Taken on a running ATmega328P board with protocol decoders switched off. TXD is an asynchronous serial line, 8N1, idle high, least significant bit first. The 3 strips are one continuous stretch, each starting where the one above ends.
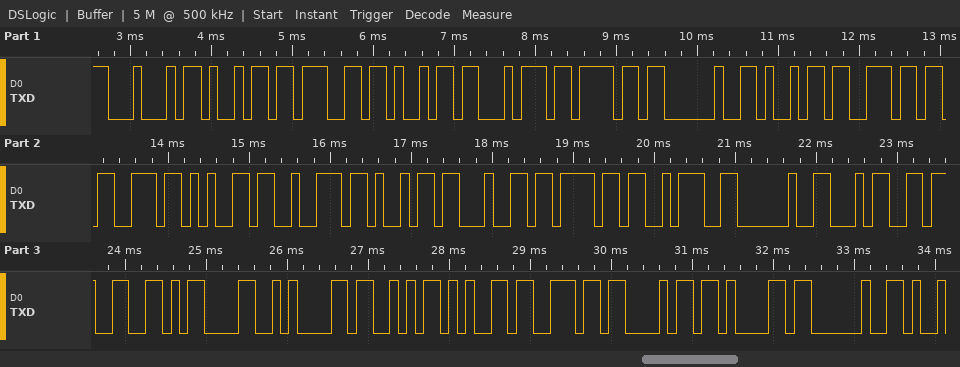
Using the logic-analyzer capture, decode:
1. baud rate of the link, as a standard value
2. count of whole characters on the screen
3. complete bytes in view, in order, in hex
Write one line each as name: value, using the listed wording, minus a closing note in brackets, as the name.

baud rate of the link, as a standard value: 9600 baud
count of whole characters on the screen: 27
complete bytes in view, in order, in hex: 44 69 67 69 74 6F 20 69 6E 73 65 72 69 64 6F 3A 20 34 33 0D 0A 53 65 6E 68 61 20
